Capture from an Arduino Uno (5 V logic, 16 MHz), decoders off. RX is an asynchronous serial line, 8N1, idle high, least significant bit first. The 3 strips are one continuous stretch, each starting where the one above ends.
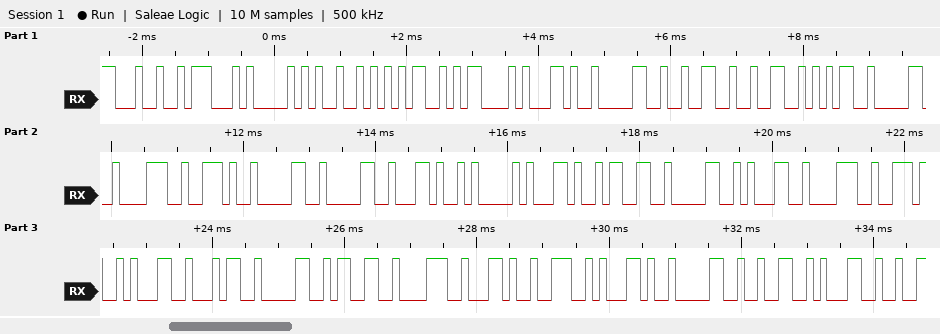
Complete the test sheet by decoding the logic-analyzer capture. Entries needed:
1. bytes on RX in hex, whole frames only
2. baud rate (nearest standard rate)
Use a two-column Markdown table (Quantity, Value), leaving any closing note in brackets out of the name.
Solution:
| Quantity | Value |
|---|---|
| bytes on RX in hex, whole frames only | 24 47 50 52 4D 43 2C 30 32 32 35 30 38 2E 30 30 2C 41 2C 33 30 31 38 2E 31 34 30 33 38 2C 4E 2C 30 32 31 |
| baud rate | 9600 baud |
